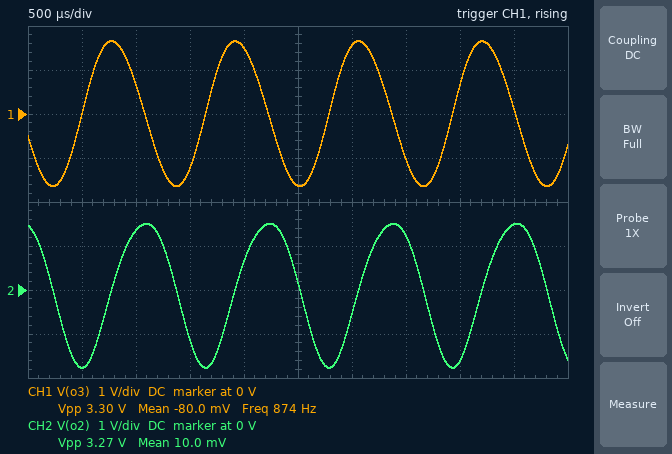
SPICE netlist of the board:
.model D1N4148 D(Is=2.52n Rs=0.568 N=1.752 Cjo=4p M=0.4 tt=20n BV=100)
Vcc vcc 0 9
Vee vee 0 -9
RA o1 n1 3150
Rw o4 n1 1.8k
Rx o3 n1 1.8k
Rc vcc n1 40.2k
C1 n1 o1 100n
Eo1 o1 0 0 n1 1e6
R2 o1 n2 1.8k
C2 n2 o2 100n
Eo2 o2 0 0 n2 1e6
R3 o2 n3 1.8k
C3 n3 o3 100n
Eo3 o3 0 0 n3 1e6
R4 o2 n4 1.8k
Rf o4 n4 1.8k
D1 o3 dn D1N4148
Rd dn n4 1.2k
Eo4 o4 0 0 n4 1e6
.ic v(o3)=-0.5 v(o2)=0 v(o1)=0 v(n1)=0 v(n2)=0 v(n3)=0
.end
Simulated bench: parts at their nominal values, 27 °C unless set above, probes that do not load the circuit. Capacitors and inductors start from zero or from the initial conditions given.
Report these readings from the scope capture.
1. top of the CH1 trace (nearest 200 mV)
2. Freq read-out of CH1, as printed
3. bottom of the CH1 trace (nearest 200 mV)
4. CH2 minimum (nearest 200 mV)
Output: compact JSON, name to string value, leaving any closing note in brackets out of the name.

{"top of the CH1 trace": "1.6 V", "Freq read-out of CH1, as printed": "874 Hz", "bottom of the CH1 trace": "-1.6 V", "CH2 minimum": "-1.8 V"}
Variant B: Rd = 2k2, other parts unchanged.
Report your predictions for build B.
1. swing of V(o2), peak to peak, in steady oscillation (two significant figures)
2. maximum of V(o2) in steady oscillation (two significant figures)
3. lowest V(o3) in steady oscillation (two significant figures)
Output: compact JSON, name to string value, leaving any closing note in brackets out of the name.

{"swing of V(o2), peak to peak, in steady oscillation": "8.6 V", "maximum of V(o2) in steady oscillation": "4.1 V", "lowest V(o3) in steady oscillation": "-3.5 V"}
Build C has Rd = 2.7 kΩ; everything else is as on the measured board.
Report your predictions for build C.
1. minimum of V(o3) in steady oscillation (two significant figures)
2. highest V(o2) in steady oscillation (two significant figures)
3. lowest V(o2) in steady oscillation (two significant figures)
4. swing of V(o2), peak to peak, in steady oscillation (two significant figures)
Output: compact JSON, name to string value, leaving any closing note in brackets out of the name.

{"minimum of V(o3) in steady oscillation": "-13 V", "highest V(o2) in steady oscillation": "17 V", "lowest V(o2) in steady oscillation": "-18 V", "swing of V(o2), peak to peak, in steady oscillation": "35 V"}
